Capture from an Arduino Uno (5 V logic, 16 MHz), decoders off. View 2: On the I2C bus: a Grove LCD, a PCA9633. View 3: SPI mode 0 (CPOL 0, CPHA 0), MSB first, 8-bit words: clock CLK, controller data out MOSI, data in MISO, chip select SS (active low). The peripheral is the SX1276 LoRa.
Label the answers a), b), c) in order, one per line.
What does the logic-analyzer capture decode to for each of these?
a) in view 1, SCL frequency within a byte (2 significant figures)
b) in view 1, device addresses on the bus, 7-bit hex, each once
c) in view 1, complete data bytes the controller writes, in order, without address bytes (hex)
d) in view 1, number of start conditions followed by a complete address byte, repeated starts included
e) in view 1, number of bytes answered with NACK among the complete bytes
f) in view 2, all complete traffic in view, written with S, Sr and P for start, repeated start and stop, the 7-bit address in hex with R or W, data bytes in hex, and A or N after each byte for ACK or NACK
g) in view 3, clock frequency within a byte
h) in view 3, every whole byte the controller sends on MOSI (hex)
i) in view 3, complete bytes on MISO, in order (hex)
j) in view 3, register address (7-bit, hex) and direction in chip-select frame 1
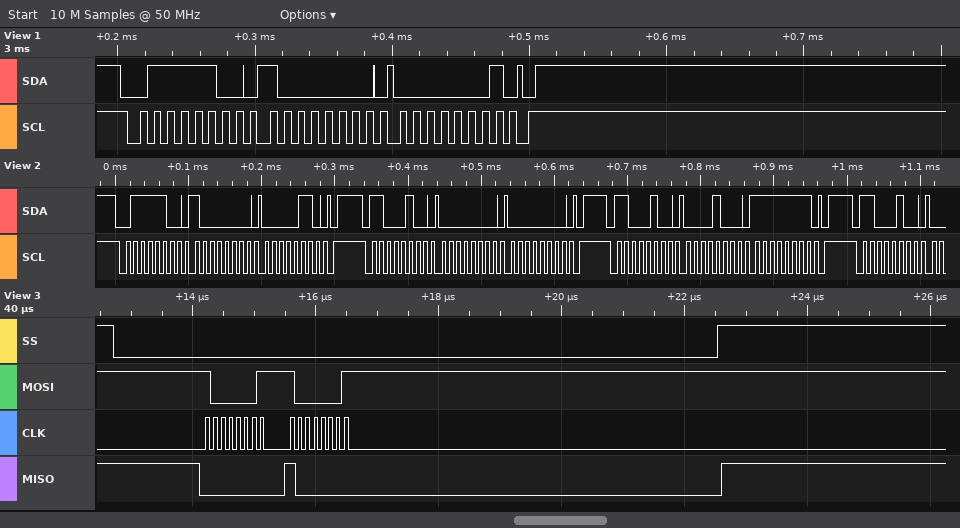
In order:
a) 100 kHz
b) 0x3E
c) 80 01
d) 1
e) 0
f) S 3EW A 80 A 06 A P S 62W A 00 A 00 A P S 62W A 08 A FF A P S 62W A
g) 8 MHz
h) 81 81
i) 00 80
j) 0x01 write
